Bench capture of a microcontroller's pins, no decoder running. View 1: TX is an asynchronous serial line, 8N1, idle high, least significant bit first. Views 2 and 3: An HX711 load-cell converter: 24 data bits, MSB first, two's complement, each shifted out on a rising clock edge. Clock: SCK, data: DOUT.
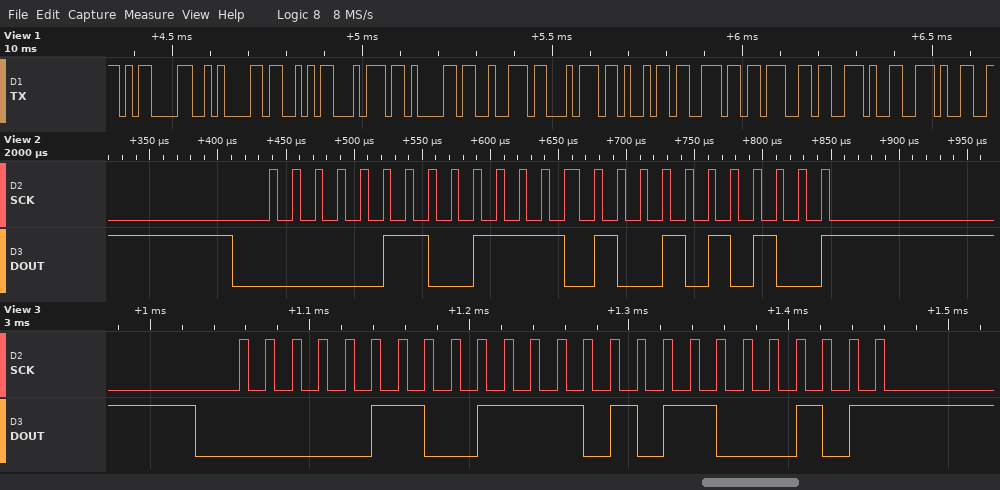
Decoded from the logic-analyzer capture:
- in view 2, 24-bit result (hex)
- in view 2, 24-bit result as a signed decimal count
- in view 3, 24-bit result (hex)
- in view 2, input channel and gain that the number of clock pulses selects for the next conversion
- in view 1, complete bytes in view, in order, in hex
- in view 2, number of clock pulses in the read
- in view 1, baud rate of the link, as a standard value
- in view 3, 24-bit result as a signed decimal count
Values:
0x067A54
424532
0x067AC5
channel A, gain 128
0x0D 0x0A 0x53 0x74 0x61 0x72 0x74 0x69 0x6E 0x67 0x2E 0x2E
25
57600 baud
424645
